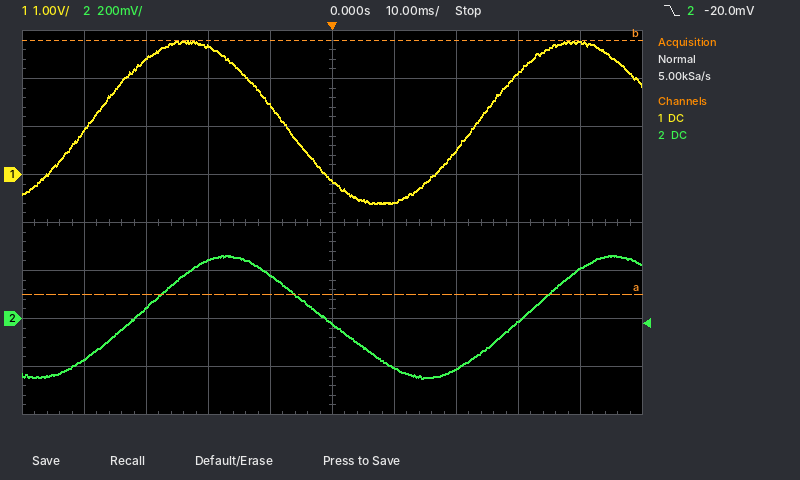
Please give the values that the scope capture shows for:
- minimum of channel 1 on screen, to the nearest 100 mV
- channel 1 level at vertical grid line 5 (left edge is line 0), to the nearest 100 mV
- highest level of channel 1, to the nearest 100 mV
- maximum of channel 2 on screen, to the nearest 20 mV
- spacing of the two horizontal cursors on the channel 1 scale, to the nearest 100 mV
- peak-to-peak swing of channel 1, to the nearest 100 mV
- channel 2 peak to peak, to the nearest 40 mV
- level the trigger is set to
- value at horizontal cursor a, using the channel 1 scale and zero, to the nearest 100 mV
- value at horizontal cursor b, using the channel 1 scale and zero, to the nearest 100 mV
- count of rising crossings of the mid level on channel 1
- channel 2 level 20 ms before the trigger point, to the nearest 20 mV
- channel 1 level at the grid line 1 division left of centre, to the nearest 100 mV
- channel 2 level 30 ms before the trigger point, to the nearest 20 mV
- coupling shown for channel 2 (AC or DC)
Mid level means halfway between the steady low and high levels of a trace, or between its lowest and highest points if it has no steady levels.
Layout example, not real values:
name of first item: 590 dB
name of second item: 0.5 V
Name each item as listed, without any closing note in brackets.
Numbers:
minimum of channel 1 on screen, to the nearest 100 mV: -600 mV
channel 1 level at vertical grid line 5 (left edge is line 0), to the nearest 100 mV: -100 mV
highest level of channel 1, to the nearest 100 mV: 2.8 V
maximum of channel 2 on screen, to the nearest 20 mV: 260 mV
spacing of the two horizontal cursors on the channel 1 scale, to the nearest 100 mV: 5.3 V
peak-to-peak swing of channel 1, to the nearest 100 mV: 3.4 V
channel 2 peak to peak, to the nearest 40 mV: 520 mV
level the trigger is set to: -20.0 mV
value at horizontal cursor a, using the channel 1 scale and zero, to the nearest 100 mV: -2.5 V
value at horizontal cursor b, using the channel 1 scale and zero, to the nearest 100 mV: 2.8 V
count of rising crossings of the mid level on channel 1: 2
channel 2 level 20 ms before the trigger point, to the nearest 20 mV: 240 mV
channel 1 level at the grid line 1 division left of centre, to the nearest 100 mV: 1.4 V
channel 2 level 30 ms before the trigger point, to the nearest 20 mV: 40 mV
coupling shown for channel 2: DC
